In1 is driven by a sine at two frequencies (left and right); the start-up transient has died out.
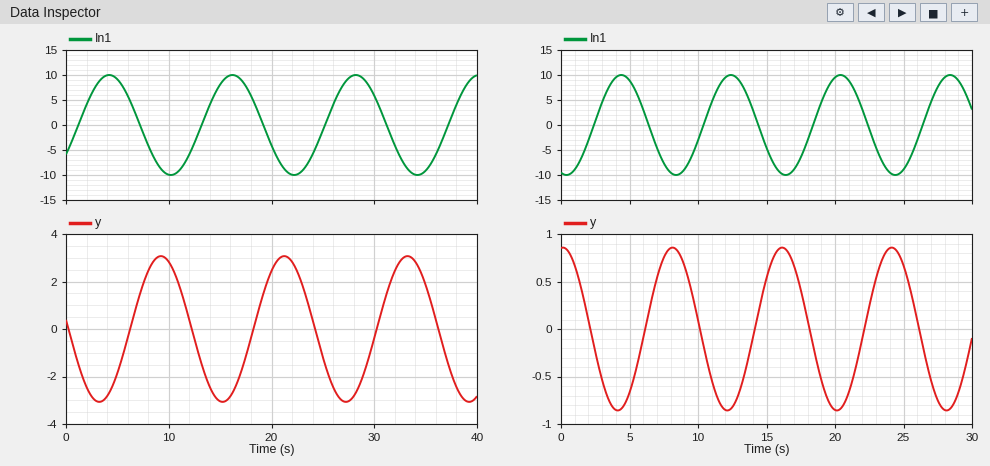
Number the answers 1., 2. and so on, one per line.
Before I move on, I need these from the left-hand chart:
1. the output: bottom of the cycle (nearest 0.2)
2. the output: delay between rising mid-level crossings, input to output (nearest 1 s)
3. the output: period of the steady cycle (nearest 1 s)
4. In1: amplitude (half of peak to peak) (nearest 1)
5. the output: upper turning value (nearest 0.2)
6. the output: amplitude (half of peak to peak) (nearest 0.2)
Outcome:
1. -3.0
2. 5 s
3. 12 s
4. 10
5. 3.0
6. 3.0
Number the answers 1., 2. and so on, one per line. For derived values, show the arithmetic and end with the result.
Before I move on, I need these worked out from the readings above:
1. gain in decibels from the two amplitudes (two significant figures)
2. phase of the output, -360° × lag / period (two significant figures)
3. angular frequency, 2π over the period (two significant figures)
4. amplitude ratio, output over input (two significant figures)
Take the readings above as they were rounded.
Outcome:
1. 20 log10(3 / 10) = -10 dB
2. -360 × 5 / 12 = -150°
3. 2π / 12 = 0.52 rad/s
4. 3 / 10 = 0.30
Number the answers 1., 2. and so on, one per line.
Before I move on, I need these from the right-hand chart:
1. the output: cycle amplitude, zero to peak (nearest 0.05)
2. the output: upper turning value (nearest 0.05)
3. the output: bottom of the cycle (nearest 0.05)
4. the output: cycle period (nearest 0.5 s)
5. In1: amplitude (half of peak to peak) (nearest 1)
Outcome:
1. 0.85
2. 0.85
3. -0.85
4. 8.0 s
5. 10
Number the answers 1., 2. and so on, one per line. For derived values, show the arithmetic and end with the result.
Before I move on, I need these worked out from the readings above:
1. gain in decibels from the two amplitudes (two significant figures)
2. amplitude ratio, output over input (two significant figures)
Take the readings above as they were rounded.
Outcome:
1. 20 log10(0.85 / 10) = -21 dB
2. 0.85 / 10 = 0.085
